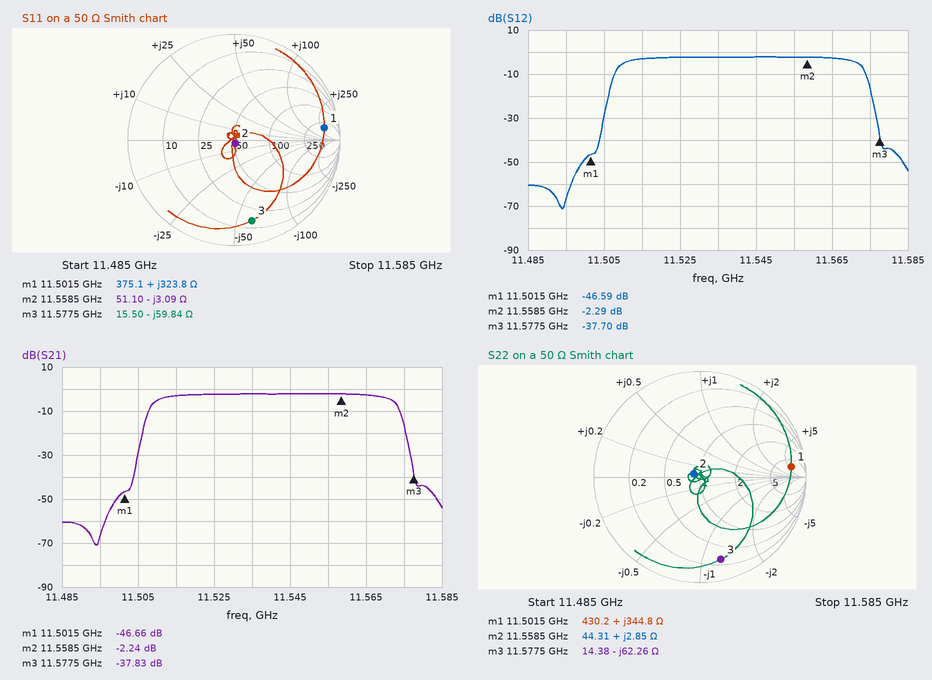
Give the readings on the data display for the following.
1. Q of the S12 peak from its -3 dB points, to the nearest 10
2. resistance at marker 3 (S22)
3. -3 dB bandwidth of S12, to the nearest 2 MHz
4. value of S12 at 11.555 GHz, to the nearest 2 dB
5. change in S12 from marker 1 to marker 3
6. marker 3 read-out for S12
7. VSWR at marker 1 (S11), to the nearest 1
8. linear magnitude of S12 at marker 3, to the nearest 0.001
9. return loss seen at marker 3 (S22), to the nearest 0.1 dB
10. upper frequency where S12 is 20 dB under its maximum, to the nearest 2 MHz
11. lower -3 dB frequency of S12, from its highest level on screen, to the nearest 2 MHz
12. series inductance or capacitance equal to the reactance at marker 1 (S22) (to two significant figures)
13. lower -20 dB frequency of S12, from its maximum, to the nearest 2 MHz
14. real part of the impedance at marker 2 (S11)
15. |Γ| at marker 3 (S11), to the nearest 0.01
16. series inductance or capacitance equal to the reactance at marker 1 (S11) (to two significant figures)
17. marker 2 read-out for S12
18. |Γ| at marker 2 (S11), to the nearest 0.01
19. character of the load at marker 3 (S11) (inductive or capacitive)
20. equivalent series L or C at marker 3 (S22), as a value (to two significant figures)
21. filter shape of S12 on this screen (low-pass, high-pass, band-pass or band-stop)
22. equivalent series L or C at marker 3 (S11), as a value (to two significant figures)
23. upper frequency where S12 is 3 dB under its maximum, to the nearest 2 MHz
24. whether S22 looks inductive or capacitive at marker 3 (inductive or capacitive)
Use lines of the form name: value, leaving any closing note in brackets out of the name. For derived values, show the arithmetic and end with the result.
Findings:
Q of the S12 peak from its -3 dB points, to the nearest 10: 11.541 GHz / 62 MHz ≈ 186, so 190 to the nearest 10
resistance at marker 3: 14.38 Ω
-3 dB bandwidth of S12, to the nearest 2 MHz: 11.572 GHz − 11.510 GHz = 62 MHz
value of S12 at 11.555 GHz, to the nearest 2 dB: -2 dB
change in S12 from marker 1 to marker 3: -37.7 − (-46.59) = 8.89 dB
marker 3 read-out for S12: -37.70 dB
VSWR at marker 1 (S11), to the nearest 1: 13
linear magnitude of S12 at marker 3, to the nearest 0.001: 10^(-37.7/20) ≈ 0.013
return loss seen at marker 3 (S22), to the nearest 0.1 dB: 1.9 dB
upper frequency where S12 is 20 dB under its maximum, to the nearest 2 MHz: 11.576 GHz
lower -3 dB frequency of S12, from its highest level on screen, to the nearest 2 MHz: 11.510 GHz
series inductance or capacitance equal to the reactance at marker 1 (S22): L = 344.8 Ω/(2π × 11.5015 GHz) ≈ 4.8 nH
lower -20 dB frequency of S12, from its maximum, to the nearest 2 MHz: 11.506 GHz
real part of the impedance at marker 2: 51.10 Ω
|Γ| at marker 3 (S11), to the nearest 0.01: 0.78
series inductance or capacitance equal to the reactance at marker 1 (S11): L = 323.8 Ω/(2π × 11.5015 GHz) ≈ 4.5 nH
marker 2 read-out for S12: -2.29 dB
|Γ| at marker 2 (S11), to the nearest 0.01: 0.03
character of the load at marker 3 (S11): capacitive
equivalent series L or C at marker 3 (S22), as a value: C = 1/(2π × 11.5775 GHz × 62.26 Ω) ≈ 221 fF, so 220 fF to two significant figures
filter shape of S12 on this screen: band-pass
equivalent series L or C at marker 3 (S11), as a value: C = 1/(2π × 11.5775 GHz × 59.84 Ω) ≈ 230 fF
upper frequency where S12 is 3 dB under its maximum, to the nearest 2 MHz: 11.572 GHz
whether S22 looks inductive or capacitive at marker 3: capacitive
